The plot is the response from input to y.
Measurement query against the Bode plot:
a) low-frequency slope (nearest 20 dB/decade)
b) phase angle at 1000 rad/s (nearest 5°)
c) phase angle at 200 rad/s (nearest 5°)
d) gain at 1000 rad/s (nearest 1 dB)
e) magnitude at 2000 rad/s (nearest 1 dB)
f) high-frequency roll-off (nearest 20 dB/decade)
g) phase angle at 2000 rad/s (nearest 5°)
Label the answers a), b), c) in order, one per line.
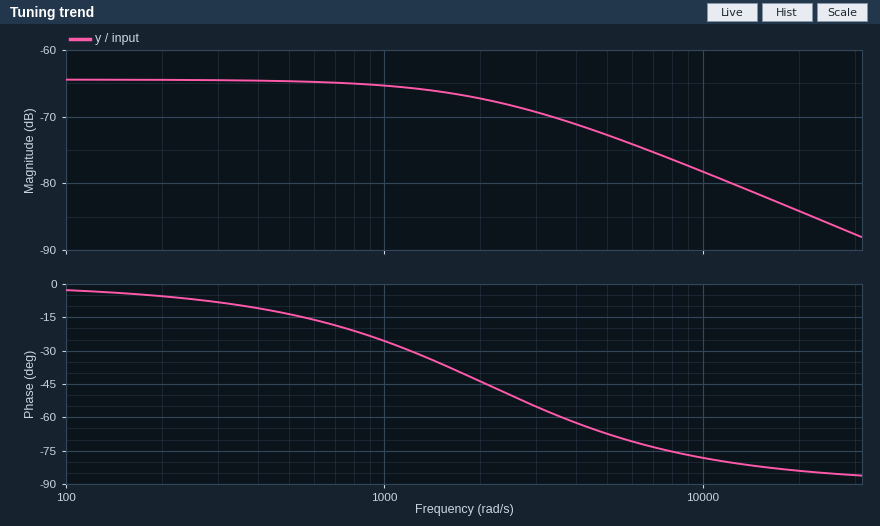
a) 0 dB/decade
b) -25°
c) -5°
d) -65 dB
e) -67 dB
f) -20 dB/decade
g) -45°
